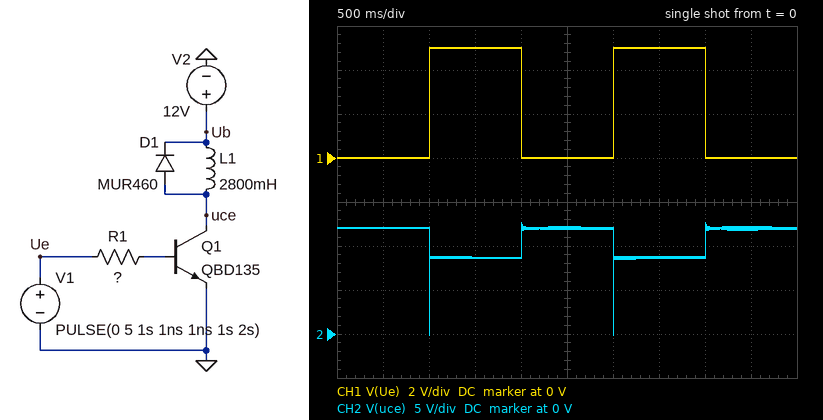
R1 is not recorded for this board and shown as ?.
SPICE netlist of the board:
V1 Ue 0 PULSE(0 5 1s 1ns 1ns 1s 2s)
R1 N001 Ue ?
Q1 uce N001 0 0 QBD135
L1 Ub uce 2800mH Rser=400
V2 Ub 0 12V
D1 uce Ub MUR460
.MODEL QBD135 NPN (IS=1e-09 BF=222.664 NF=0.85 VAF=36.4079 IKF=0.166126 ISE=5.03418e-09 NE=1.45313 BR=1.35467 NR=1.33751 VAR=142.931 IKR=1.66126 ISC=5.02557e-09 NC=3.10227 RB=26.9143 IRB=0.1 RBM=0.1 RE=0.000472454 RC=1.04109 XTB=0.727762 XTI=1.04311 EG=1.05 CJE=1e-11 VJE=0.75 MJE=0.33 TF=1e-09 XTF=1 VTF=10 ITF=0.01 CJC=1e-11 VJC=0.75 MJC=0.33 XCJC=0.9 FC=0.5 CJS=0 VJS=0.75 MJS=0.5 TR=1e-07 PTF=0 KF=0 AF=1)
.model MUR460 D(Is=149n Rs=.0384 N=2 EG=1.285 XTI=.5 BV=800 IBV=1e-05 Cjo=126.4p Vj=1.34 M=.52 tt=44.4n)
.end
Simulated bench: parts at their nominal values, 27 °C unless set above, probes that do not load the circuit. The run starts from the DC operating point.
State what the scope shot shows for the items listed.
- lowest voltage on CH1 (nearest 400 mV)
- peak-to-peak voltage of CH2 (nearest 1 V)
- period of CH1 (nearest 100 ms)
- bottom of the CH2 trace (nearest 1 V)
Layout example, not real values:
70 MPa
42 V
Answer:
0 V
13 V
2.0 s
0 V
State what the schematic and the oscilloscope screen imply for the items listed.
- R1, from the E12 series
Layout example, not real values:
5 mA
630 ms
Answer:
56 kΩ
